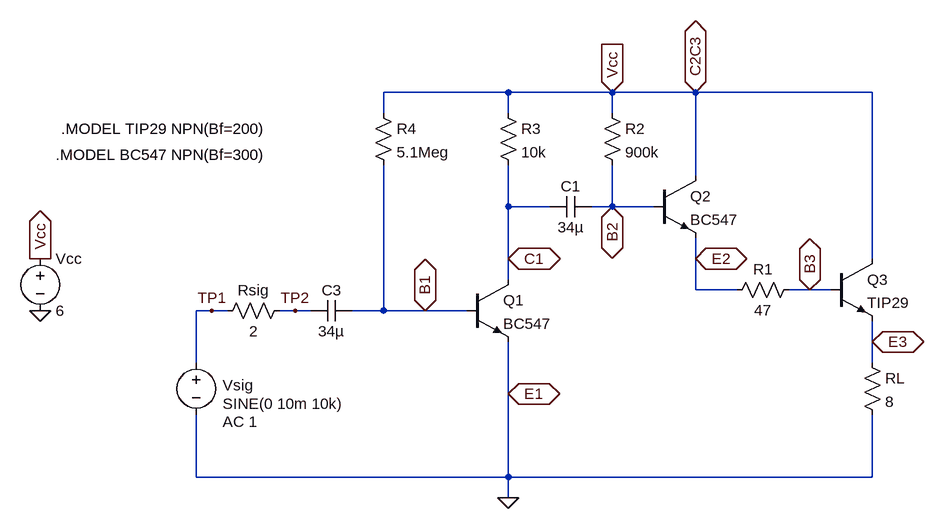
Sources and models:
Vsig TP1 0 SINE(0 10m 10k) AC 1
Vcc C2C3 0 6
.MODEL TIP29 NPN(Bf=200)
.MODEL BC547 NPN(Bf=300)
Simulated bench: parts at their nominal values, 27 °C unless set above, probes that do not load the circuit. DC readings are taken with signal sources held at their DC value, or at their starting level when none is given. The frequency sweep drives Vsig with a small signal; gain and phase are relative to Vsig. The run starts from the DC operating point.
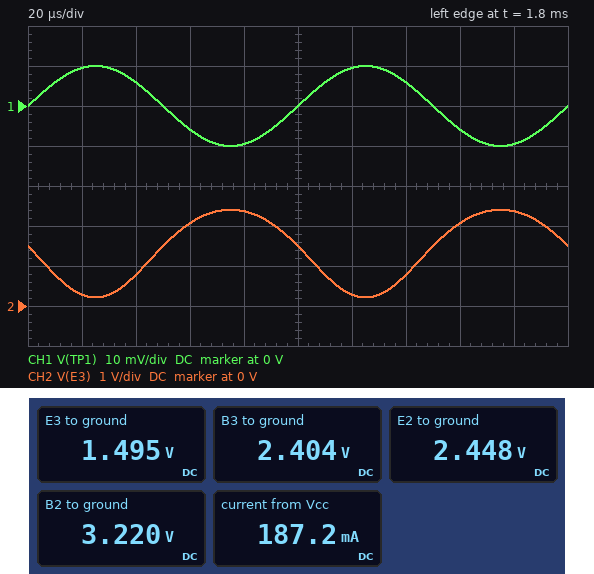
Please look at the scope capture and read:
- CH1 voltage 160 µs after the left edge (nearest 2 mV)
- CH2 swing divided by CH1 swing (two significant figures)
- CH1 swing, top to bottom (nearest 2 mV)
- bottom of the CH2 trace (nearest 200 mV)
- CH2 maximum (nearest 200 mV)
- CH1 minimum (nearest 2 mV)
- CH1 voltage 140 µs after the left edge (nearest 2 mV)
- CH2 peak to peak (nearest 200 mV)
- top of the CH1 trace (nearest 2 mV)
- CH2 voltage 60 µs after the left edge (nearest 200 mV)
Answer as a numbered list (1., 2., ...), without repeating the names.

1. -6 mV
2. 110
3. 20 mV
4. 200 mV
5. 2.4 V
6. -10 mV
7. 6 mV
8. 2.2 V
9. 10 mV
10. 2.0 V
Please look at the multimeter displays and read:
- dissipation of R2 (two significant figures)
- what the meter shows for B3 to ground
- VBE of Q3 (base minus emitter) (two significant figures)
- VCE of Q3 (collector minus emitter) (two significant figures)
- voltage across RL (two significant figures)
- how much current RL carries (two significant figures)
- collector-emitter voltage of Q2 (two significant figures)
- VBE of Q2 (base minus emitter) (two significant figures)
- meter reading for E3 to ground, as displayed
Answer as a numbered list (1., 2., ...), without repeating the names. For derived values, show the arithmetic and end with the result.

1. (6 V - 3.22 V)^2 / 900 kΩ = 8.6 µW
2. 2.404 V
3. 2.404 V - 1.495 V = 910 mV
4. 6 V - 1.495 V = 4.5 V
5. 1.495 V = 1.5 V
6. (1.495 V) / 8 Ω = 190 mA
7. 6 V - 2.448 V = 3.6 V
8. 3.22 V - 2.448 V = 770 mV
9. 1.495 V
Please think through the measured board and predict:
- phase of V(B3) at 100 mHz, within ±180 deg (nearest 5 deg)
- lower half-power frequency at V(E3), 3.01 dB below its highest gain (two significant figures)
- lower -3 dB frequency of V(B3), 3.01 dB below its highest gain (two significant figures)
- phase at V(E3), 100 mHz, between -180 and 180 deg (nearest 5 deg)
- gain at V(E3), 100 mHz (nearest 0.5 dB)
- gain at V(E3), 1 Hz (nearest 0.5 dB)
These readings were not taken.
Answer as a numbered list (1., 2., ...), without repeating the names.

1. -110 deg
2. 190 mHz
3. 190 mHz
4. -110 deg
5. 34.0 dB
6. 40.5 dB
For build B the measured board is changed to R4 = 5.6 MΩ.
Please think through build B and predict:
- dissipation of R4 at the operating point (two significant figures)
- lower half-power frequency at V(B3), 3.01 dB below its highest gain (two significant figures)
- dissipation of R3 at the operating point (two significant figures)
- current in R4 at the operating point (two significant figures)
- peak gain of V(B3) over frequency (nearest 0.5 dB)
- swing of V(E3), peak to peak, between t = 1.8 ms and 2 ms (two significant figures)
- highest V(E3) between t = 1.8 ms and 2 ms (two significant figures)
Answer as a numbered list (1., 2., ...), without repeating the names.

1. 4.9 µW
2. 170 mHz
3. 790 µW
4. 940 nA
5. 40.0 dB
6. 2.0 V
7. 2.3 V
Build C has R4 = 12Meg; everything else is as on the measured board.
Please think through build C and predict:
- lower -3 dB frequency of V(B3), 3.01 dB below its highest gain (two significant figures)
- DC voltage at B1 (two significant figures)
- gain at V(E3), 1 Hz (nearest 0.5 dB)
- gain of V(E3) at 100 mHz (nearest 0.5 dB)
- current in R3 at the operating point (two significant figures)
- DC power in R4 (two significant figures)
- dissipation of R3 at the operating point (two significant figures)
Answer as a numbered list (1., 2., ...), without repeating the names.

1. 82 mHz
2. 720 mV
3. 33.5 dB
4. 31.0 dB
5. 130 µA
6. 2.3 µW
7. 170 µW
